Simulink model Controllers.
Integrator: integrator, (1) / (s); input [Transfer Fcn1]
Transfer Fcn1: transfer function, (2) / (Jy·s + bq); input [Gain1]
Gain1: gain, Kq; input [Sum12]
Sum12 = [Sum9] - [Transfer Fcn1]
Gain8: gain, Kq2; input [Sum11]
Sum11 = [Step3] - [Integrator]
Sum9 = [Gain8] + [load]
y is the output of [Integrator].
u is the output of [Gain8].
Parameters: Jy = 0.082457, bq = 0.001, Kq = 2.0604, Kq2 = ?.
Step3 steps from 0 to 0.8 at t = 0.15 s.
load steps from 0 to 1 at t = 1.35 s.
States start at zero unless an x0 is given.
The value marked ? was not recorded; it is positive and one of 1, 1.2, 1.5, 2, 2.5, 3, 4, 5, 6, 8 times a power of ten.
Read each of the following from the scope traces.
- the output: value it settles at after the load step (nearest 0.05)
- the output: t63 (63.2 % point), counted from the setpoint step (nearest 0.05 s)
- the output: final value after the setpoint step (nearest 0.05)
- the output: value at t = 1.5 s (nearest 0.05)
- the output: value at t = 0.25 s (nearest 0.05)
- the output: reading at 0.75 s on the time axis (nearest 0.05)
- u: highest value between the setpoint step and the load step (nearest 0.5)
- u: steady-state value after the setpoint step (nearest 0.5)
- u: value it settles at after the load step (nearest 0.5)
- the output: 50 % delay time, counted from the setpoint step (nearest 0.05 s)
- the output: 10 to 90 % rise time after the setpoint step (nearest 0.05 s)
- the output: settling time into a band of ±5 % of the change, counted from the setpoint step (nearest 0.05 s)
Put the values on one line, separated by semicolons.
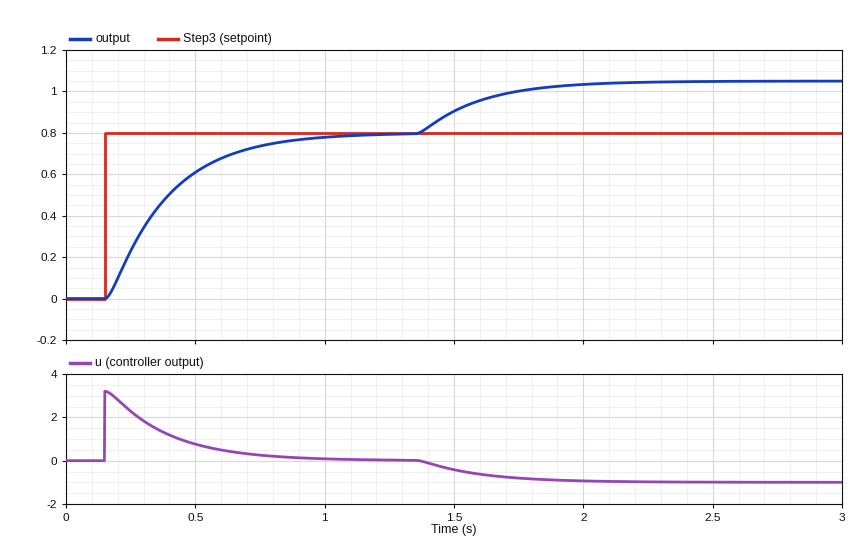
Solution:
1.05; 0.25 s; 0.80; 0.90; 0.25; 0.75; 3.0; 0.0; -1.0; 0.20 s; 0.50 s; 0.70 s
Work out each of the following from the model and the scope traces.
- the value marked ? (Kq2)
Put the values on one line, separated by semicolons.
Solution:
4
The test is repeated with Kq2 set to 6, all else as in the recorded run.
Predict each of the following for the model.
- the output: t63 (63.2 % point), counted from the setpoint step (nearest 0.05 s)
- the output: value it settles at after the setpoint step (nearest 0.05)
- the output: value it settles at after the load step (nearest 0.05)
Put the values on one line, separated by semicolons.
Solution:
0.15 s; 0.80; 0.95
